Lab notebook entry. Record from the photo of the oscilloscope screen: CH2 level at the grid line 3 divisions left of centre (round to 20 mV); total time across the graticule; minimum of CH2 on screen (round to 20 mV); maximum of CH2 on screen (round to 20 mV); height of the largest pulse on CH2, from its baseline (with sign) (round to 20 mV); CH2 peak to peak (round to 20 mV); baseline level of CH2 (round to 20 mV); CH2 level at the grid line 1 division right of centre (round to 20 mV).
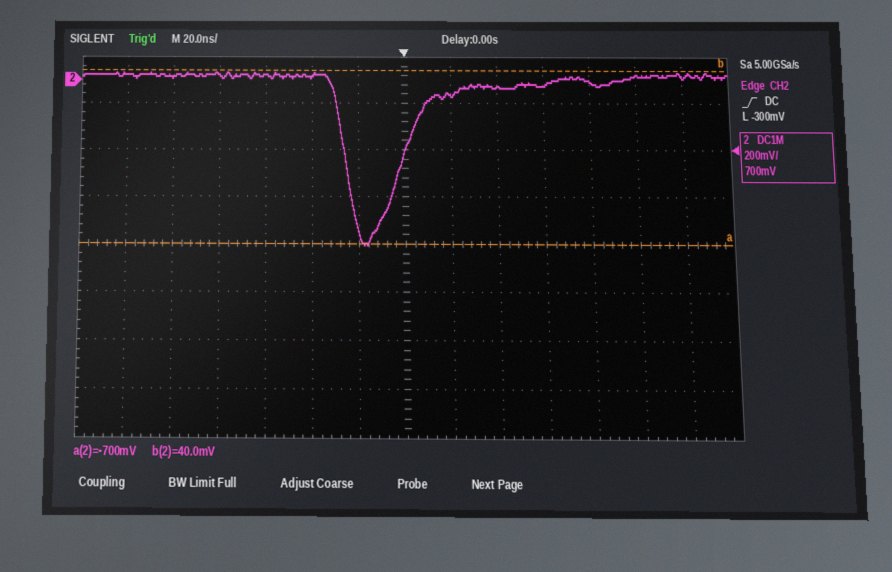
20 mV
280 ns
-700 mV
40 mV
-720 mV
740 mV
20 mV
-60 mV
